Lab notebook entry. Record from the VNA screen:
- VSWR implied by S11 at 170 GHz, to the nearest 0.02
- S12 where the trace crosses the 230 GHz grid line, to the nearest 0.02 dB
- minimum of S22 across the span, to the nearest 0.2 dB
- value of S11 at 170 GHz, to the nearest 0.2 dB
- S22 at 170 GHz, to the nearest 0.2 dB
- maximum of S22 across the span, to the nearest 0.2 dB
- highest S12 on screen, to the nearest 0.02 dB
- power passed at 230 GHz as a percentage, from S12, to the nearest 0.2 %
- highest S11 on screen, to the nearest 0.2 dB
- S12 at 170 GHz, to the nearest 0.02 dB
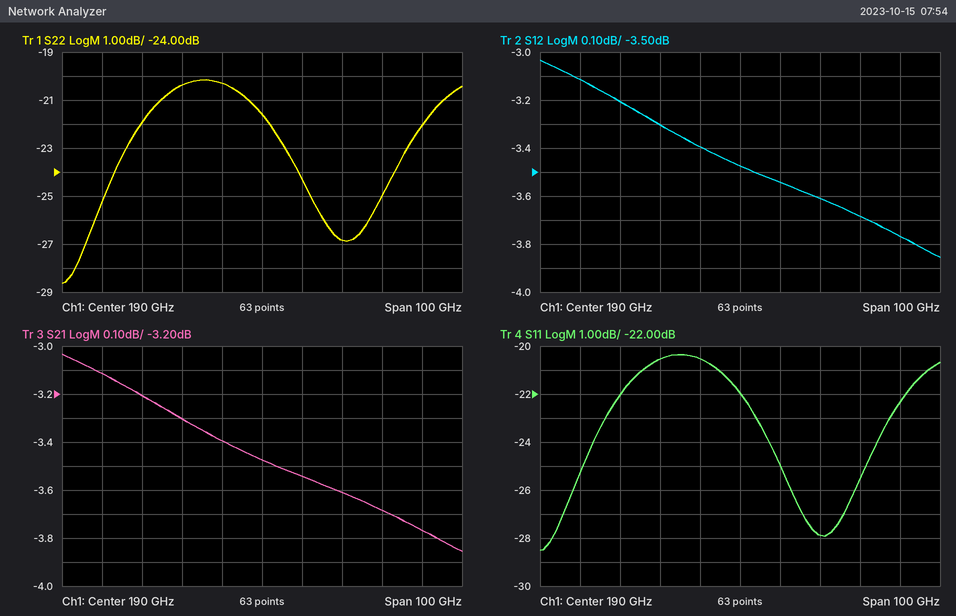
1.20
-3.76 dB
-28.6 dB
-20.6 dB
-20.4 dB
-20.2 dB
-3.04 dB
42.0 %
-20.4 dB
-3.30 dB
